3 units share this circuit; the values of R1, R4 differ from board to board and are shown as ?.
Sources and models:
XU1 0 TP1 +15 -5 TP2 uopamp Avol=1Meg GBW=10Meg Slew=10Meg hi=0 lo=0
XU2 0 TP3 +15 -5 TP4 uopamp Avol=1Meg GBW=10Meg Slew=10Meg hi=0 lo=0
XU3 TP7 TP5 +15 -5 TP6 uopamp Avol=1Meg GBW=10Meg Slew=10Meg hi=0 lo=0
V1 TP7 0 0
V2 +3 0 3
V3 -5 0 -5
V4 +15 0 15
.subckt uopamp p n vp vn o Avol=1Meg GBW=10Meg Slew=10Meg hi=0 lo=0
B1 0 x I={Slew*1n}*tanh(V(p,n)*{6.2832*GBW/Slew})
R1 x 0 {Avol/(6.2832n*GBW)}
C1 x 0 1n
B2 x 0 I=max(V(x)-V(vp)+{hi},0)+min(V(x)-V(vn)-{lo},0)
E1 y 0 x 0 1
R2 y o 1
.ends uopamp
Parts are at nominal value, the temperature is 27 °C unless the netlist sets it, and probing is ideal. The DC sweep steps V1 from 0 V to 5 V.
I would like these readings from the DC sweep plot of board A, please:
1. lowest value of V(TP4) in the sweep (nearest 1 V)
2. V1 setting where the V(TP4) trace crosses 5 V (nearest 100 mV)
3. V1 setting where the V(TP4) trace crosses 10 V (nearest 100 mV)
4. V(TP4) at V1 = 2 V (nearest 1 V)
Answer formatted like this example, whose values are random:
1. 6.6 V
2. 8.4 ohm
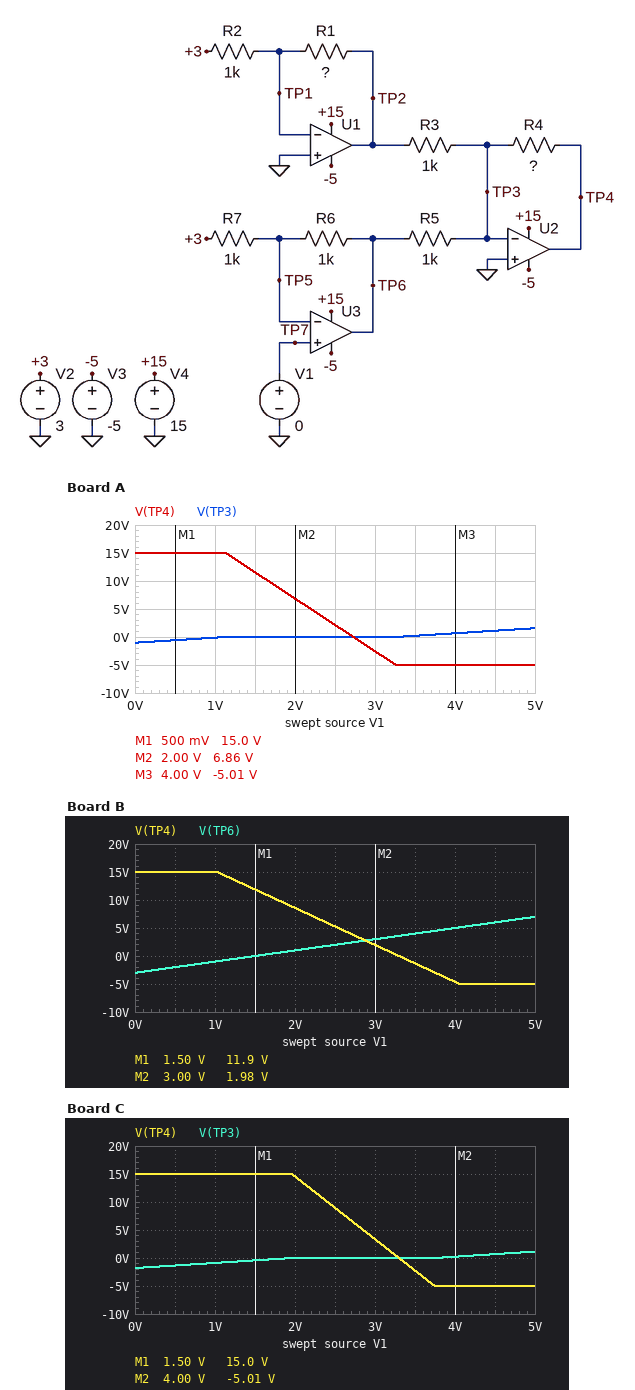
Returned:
1. -5 V
2. 2.2 V
3. 1.7 V
4. 7 V
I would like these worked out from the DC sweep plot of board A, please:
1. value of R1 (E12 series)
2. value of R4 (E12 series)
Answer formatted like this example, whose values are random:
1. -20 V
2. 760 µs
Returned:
1. 820 Ω
2. 4.7 kΩ
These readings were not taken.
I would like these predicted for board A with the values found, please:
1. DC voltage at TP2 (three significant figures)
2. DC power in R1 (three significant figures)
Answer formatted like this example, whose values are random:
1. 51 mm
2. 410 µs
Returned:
1. -2.46 V
2. 7.38 mW
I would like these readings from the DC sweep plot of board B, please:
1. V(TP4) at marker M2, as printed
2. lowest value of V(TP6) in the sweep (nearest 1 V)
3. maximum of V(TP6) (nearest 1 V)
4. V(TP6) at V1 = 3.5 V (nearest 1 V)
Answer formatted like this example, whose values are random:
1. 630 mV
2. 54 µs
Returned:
1. 1.98 V
2. -3 V
3. 7 V
4. 4 V
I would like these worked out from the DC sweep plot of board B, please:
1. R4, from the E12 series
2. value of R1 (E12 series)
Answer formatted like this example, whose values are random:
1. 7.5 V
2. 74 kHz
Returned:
1. 3.3 kΩ
2. 1.2 kΩ
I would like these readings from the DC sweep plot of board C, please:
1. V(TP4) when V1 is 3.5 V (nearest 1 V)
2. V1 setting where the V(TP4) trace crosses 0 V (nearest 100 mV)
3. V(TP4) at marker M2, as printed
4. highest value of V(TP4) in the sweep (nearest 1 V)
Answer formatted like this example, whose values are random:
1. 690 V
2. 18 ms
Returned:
1. -2 V
2. 3.3 V
3. -5.01 V
4. 15 V
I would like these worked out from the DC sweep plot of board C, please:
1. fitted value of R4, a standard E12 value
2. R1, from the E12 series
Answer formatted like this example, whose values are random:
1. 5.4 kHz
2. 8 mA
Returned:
1. 5.6 kΩ
2. 1.2 kΩ
